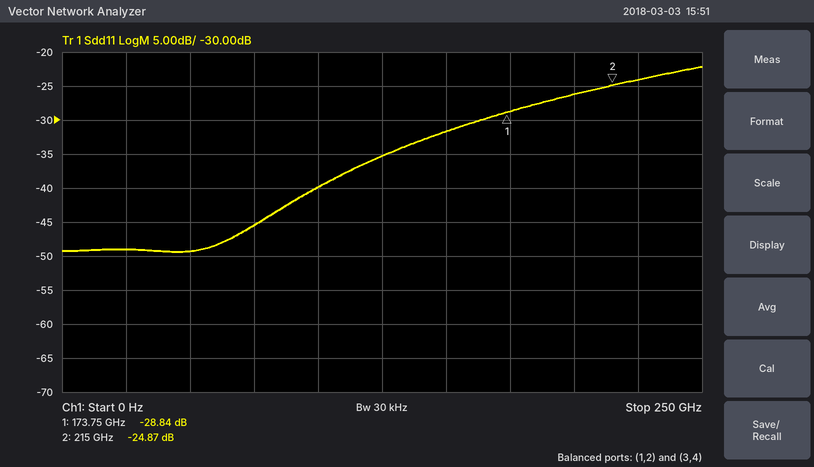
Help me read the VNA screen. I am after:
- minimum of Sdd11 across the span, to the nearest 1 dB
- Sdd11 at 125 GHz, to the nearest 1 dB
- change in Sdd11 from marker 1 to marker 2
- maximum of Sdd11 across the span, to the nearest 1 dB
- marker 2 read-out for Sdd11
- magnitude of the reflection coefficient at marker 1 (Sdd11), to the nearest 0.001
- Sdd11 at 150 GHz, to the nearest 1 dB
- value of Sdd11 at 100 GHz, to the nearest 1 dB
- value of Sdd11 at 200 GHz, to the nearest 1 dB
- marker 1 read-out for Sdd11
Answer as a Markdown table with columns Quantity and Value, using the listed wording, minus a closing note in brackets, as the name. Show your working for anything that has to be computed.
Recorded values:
| Quantity | Value |
|---|---|
| minimum of Sdd11 across the span, to the nearest 1 dB | -49 dB |
| Sdd11 at 125 GHz, to the nearest 1 dB | -35 dB |
| change in Sdd11 from marker 1 to marker 2 | -24.87 − (-28.84) = 3.97 dB |
| maximum of Sdd11 across the span, to the nearest 1 dB | -22 dB |
| marker 2 read-out for Sdd11 | -24.87 dB |
| magnitude of the reflection coefficient at marker 1 (Sdd11), to the nearest 0.001 | 10^(-28.84/20) ≈ 0.036 |
| Sdd11 at 150 GHz, to the nearest 1 dB | -32 dB |
| value of Sdd11 at 100 GHz, to the nearest 1 dB | -40 dB |
| value of Sdd11 at 200 GHz, to the nearest 1 dB | -26 dB |
| marker 1 read-out for Sdd11 | -28.84 dB |
